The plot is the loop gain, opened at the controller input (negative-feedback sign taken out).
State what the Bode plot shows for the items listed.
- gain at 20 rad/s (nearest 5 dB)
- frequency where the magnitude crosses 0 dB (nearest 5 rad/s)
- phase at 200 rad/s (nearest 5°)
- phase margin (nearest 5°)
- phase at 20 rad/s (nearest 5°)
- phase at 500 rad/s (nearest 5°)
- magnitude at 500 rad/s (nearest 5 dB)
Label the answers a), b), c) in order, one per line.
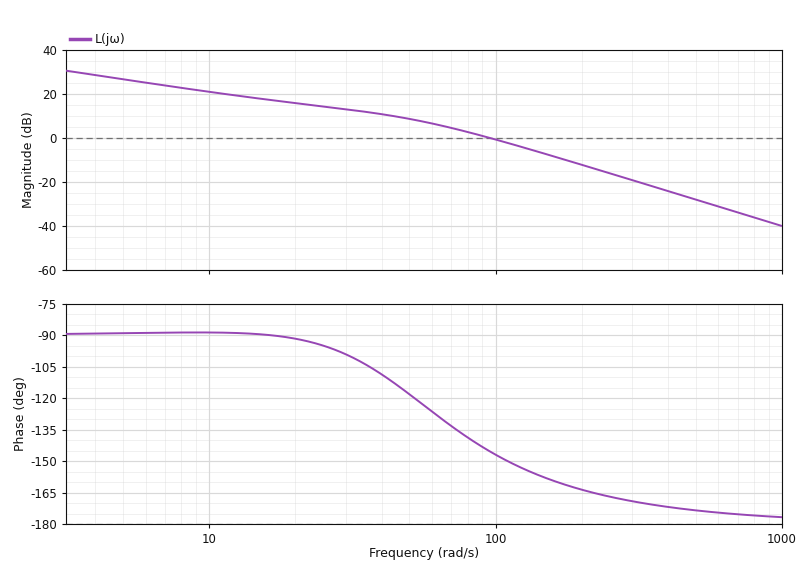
a) 15 dB
b) 95 rad/s
c) -165°
d) 35°
e) -90°
f) -175°
g) -30 dB
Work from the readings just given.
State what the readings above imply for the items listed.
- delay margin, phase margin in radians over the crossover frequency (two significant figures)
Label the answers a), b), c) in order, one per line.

a) 0.0064 s
